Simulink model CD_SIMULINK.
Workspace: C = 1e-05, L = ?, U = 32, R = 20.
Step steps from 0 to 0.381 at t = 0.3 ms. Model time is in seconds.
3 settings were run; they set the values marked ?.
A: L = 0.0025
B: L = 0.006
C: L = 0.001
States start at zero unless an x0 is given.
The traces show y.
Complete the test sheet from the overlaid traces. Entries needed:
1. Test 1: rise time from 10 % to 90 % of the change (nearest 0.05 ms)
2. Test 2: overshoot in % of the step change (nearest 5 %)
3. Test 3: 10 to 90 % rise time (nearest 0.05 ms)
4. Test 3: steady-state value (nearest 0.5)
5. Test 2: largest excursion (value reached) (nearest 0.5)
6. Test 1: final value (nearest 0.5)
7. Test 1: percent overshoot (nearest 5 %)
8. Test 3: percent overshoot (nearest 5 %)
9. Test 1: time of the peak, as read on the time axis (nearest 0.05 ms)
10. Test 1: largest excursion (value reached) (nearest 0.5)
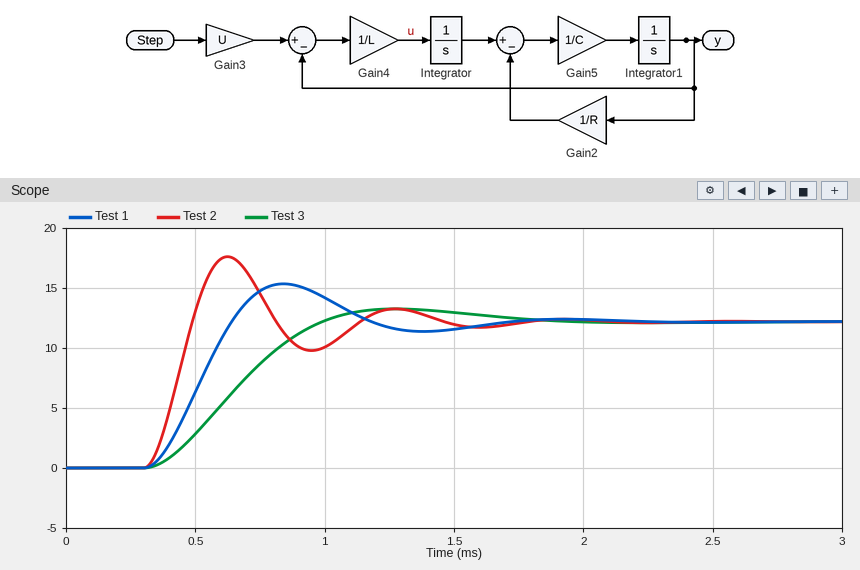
0.25 ms
45 %
0.45 ms
12.0
17.5
12.0
25 %
10 %
0.85 ms
15.5
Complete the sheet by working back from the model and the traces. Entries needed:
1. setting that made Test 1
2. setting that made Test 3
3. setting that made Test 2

A
B
C
